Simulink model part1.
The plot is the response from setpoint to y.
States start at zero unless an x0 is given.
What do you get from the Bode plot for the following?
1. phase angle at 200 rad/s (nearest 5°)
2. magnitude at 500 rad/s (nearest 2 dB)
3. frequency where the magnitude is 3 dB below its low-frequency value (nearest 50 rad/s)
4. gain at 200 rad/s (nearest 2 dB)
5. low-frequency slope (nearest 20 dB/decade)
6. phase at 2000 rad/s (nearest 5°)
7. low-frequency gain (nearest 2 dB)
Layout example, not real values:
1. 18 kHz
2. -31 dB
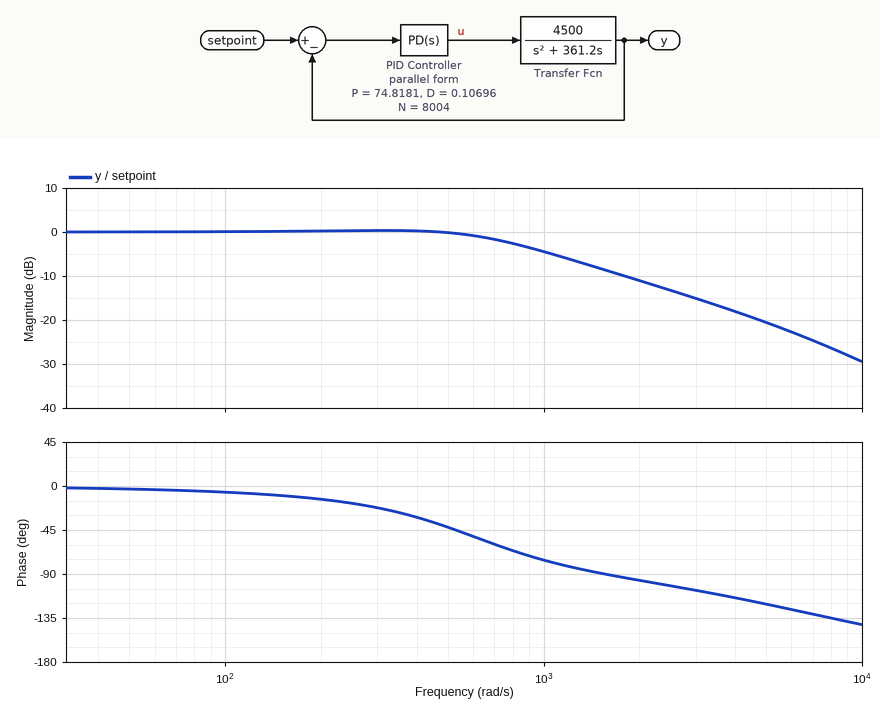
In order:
1. -15°
2. 0 dB
3. 850 rad/s
4. 0 dB
5. 0 dB/decade
6. -95°
7. 0 dB
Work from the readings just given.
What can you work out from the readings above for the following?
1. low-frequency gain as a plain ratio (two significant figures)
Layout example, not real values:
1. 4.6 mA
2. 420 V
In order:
1. 1.0
